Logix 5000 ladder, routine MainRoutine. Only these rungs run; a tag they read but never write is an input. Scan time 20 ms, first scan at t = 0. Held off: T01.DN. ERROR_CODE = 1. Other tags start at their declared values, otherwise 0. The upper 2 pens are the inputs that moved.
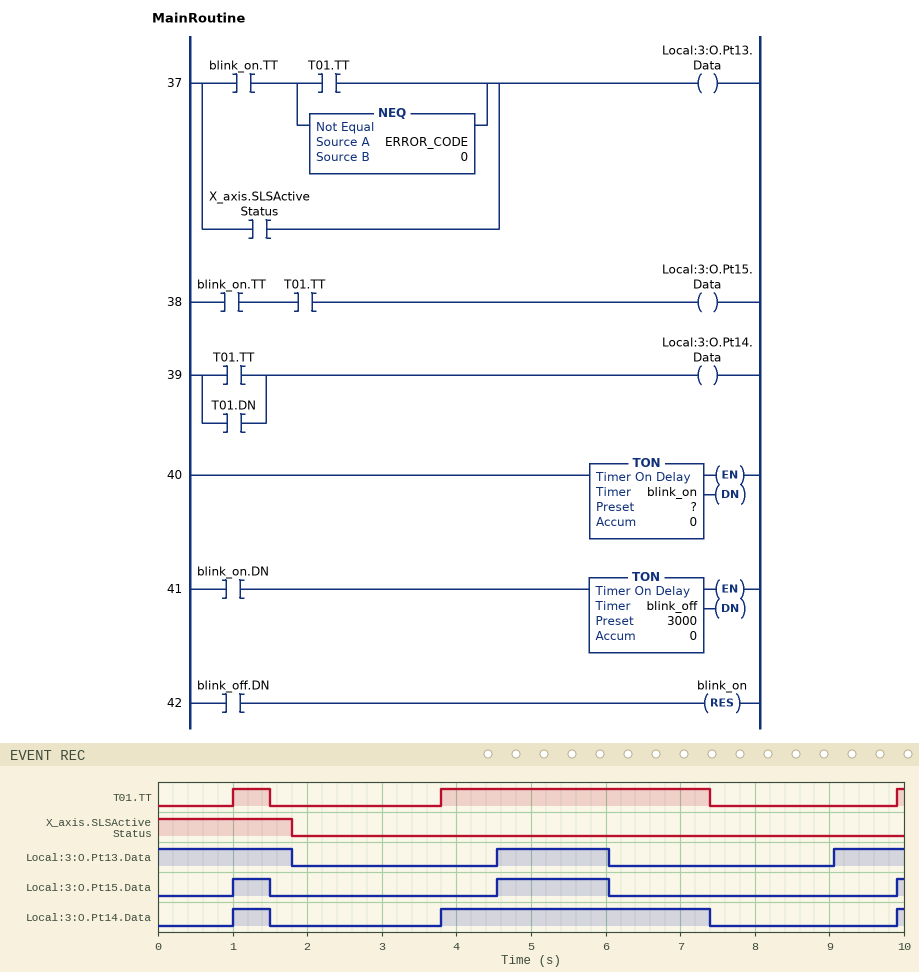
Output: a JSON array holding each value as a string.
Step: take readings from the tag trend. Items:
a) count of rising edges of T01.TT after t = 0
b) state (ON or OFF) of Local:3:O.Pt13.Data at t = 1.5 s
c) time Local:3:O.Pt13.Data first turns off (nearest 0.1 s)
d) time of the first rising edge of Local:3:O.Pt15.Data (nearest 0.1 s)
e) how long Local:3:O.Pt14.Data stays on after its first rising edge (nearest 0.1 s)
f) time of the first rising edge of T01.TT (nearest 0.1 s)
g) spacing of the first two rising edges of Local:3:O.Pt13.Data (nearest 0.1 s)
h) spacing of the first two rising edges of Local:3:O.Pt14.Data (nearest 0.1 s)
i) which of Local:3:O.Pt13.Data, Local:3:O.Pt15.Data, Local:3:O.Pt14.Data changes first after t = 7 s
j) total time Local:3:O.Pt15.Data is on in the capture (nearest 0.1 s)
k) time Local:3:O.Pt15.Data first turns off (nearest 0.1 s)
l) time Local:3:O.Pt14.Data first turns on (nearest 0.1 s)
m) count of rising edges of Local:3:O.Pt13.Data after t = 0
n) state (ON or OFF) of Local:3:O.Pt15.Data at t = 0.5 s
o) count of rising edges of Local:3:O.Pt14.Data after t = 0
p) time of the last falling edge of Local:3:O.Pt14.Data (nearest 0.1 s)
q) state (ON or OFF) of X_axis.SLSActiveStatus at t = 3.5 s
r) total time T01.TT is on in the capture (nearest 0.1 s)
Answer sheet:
["3", "ON", "1.8 s", "1.0 s", "0.5 s", "1.0 s", "4.5 s", "2.8 s", "Local:3:O.Pt14.Data", "2.1 s", "1.5 s", "1.0 s", "2", "OFF", "3", "7.4 s", "OFF", "4.2 s"]
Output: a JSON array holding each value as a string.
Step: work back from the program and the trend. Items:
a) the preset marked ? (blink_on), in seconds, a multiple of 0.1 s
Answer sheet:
["1.5 s"]
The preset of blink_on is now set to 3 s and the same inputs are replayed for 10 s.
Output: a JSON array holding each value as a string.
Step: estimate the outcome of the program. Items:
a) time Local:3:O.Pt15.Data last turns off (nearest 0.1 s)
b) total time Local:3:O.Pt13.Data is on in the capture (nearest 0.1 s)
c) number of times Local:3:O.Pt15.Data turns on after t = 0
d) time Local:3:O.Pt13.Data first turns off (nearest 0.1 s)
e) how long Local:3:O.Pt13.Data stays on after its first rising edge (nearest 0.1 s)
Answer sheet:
["7.4 s", "6.0 s", "2", "3.0 s", "3.0 s"]
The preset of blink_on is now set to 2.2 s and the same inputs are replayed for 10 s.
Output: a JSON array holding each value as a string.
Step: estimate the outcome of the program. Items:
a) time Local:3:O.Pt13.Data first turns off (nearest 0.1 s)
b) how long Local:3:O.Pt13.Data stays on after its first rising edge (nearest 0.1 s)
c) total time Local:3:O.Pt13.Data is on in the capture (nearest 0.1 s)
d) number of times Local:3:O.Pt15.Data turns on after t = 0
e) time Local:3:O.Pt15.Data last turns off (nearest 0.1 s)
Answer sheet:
["2.2 s", "2.2 s", "4.4 s", "2", "7.4 s"]
